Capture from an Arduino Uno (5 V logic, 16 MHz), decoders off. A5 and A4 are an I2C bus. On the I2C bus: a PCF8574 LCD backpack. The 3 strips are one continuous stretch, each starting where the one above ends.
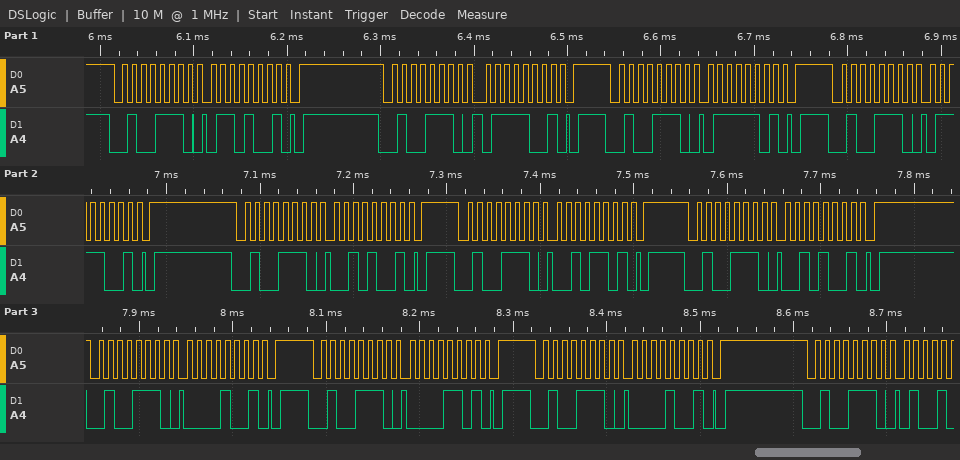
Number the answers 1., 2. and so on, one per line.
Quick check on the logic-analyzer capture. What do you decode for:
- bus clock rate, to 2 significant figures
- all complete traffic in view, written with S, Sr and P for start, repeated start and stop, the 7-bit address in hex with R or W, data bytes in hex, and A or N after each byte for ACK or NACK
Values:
1. 100 kHz
2. S 27W A 69 A P S 27W A 79 A P S 27W A 7D A P S 27W A 79 A P S 27W A 29 A P S 27W A 2D A P S 27W A 29 A P S 27W A 09 A P S 27W A 0D A P S 27W A 09 A P S 27W A
